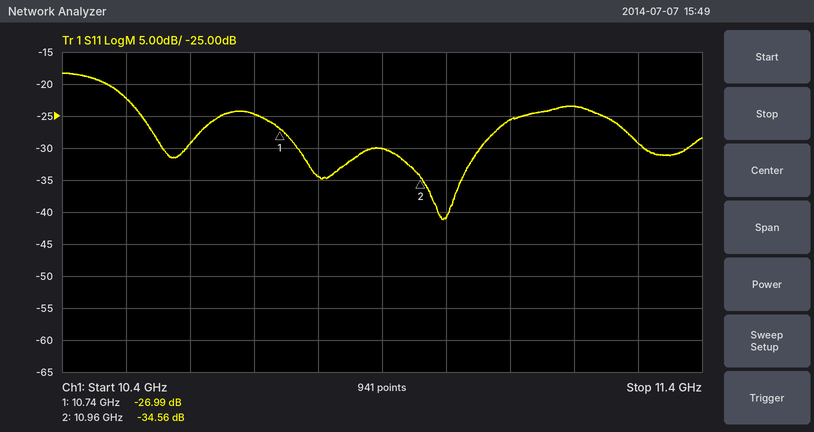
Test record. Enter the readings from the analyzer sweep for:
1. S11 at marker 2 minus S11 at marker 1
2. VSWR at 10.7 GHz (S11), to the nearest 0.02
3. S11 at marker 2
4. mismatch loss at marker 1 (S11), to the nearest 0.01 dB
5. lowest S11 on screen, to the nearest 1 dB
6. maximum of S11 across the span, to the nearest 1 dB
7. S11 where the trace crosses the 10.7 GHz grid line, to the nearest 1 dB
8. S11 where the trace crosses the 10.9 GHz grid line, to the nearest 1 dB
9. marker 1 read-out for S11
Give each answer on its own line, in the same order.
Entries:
-7.57 dB
1.12
-34.56 dB
0.01 dB
-41 dB
-18 dB
-25 dB
-30 dB
-26.99 dB
